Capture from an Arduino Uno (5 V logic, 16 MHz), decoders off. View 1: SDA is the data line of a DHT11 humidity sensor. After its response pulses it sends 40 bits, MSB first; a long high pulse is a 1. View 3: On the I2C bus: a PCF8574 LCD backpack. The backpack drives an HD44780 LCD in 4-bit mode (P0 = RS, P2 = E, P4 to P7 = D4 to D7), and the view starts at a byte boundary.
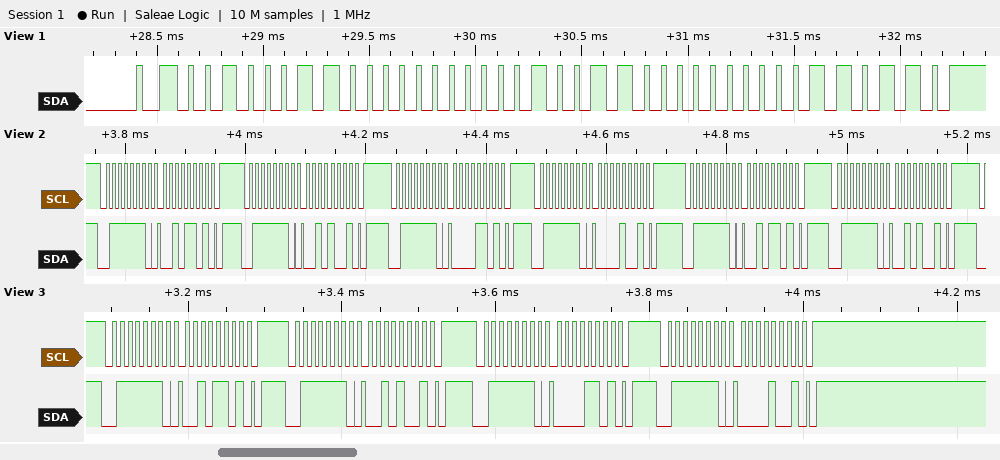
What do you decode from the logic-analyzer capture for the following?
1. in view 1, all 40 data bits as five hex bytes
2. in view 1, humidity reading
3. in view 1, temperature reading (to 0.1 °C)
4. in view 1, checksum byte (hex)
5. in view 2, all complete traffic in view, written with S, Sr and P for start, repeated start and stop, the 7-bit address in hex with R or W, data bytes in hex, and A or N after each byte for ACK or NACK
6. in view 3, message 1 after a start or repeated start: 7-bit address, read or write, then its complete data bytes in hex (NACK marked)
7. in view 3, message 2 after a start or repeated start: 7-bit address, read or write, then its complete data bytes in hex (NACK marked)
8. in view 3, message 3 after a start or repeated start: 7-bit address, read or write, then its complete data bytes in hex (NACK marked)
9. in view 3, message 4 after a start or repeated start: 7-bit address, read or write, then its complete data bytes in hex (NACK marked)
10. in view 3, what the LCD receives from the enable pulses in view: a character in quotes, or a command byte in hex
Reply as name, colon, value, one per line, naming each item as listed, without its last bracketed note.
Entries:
in view 1, all 40 data bits as five hex bytes: 23 00 13 00 36
in view 1, humidity reading: 35 %
in view 1, temperature reading: 19.0 °C
in view 1, checksum byte: 0x36
in view 2, all complete traffic in view, written with S, Sr and P for start, repeated start and stop, the 7-bit address in hex with R or W, data bytes in hex, and A or N after each byte for ACK or NACK: S 3FW A 2D A P S 3FW A 29 A P S 3FW A 0D A P S 3FW A 09 A P S 3FW A 2D A P S 3FW A 29 A P
in view 3, message 1 after a start or repeated start: 7-bit address, read or write, then its complete data bytes in hex: 0x3F write: 2D
in view 3, message 2 after a start or repeated start: 7-bit address, read or write, then its complete data bytes in hex: 0x3F write: 29
in view 3, message 3 after a start or repeated start: 7-bit address, read or write, then its complete data bytes in hex: 0x3F write: 0D
in view 3, message 4 after a start or repeated start: 7-bit address, read or write, then its complete data bytes in hex: 0x3F write: 09
in view 3, what the LCD receives from the enable pulses in view: a character in quotes, or a command byte in hex: ' '
